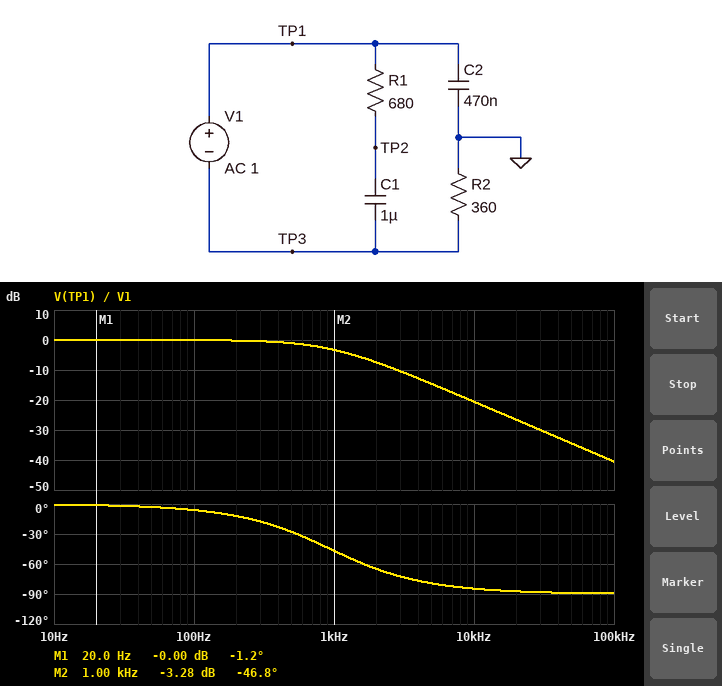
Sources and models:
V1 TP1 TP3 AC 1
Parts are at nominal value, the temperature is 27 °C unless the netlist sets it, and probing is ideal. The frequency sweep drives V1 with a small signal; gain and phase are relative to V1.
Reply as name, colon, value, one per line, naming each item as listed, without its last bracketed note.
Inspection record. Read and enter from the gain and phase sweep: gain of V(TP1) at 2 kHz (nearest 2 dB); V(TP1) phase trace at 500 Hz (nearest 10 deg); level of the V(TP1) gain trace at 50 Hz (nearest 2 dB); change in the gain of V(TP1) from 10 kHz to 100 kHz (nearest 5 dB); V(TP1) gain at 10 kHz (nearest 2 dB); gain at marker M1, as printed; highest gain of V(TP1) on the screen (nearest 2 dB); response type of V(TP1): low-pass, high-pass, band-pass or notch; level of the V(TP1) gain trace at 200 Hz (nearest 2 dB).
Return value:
gain of V(TP1) at 2 kHz: -8 dB
V(TP1) phase trace at 500 Hz: -30 deg
level of the V(TP1) gain trace at 50 Hz: 0 dB
change in the gain of V(TP1) from 10 kHz to 100 kHz: -20 dB
V(TP1) gain at 10 kHz: -20 dB
gain at marker M1, as printed: -0.00 dB
highest gain of V(TP1) on the screen: 0 dB
response type of V(TP1): low-pass, high-pass, band-pass or notch: low-pass
level of the V(TP1) gain trace at 200 Hz: 0 dB
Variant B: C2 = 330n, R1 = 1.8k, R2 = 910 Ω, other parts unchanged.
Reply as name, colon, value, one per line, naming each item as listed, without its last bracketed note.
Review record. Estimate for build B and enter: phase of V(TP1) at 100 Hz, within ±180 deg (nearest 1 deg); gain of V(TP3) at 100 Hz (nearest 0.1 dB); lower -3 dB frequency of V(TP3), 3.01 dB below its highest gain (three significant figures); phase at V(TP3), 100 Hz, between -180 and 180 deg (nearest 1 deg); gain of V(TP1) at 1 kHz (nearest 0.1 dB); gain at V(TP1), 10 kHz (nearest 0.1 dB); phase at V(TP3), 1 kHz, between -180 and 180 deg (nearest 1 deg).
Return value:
phase of V(TP1) at 100 Hz, within ±180 deg: -11 deg
gain of V(TP3) at 100 Hz: -14.6 dB
lower -3 dB frequency of V(TP3), 3.01 dB below its highest gain: 530 Hz
phase at V(TP3), 100 Hz, between -180 and 180 deg: -101 deg
gain of V(TP1) at 1 kHz: -6.6 dB
gain at V(TP1), 10 kHz: -25.5 dB
phase at V(TP3), 1 kHz, between -180 and 180 deg: -152 deg
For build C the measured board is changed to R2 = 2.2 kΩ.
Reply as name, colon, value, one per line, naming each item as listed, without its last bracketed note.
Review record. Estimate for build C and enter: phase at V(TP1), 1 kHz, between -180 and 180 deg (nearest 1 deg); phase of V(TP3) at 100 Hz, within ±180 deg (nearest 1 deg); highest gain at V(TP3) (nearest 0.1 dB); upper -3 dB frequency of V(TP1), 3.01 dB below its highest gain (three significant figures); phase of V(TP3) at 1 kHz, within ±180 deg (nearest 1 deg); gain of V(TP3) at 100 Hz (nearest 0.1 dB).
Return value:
phase at V(TP1), 1 kHz, between -180 and 180 deg: -81 deg
phase of V(TP3) at 100 Hz, within ±180 deg: -123 deg
highest gain at V(TP3): 0 dB
upper -3 dB frequency of V(TP1), 3.01 dB below its highest gain: 154 Hz
phase of V(TP3) at 1 kHz, within ±180 deg: -171 deg
gain of V(TP3) at 100 Hz: -5.3 dB
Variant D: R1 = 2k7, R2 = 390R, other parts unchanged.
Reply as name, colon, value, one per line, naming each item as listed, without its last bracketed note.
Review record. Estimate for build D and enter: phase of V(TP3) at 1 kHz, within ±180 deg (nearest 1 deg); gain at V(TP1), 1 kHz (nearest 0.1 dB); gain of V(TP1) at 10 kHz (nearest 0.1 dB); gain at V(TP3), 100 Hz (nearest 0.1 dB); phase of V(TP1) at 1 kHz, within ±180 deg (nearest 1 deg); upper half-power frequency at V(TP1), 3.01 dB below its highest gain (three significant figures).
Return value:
phase of V(TP3) at 1 kHz, within ±180 deg: -139 deg
gain at V(TP1), 1 kHz: -3.7 dB
gain of V(TP1) at 10 kHz: -21.3 dB
gain at V(TP3), 100 Hz: -18.8 dB
phase of V(TP1) at 1 kHz, within ±180 deg: -49 deg
upper half-power frequency at V(TP1), 3.01 dB below its highest gain: 868 Hz
